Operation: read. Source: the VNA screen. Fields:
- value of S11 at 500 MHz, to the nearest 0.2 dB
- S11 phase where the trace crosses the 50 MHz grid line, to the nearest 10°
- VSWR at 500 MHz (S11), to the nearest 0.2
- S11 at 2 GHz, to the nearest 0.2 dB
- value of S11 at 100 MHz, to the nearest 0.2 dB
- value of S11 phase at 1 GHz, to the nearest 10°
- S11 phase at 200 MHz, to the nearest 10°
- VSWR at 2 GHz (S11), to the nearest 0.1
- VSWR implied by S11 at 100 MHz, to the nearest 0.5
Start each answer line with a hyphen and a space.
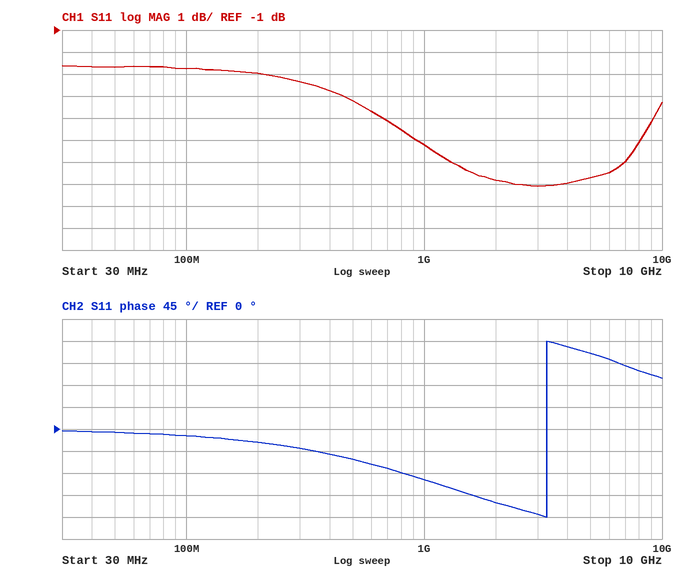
- -4.2 dB
- -10°
- 4.2
- -7.8 dB
- -2.8 dB
- -100°
- -30°
- 2.4
- 6.5
